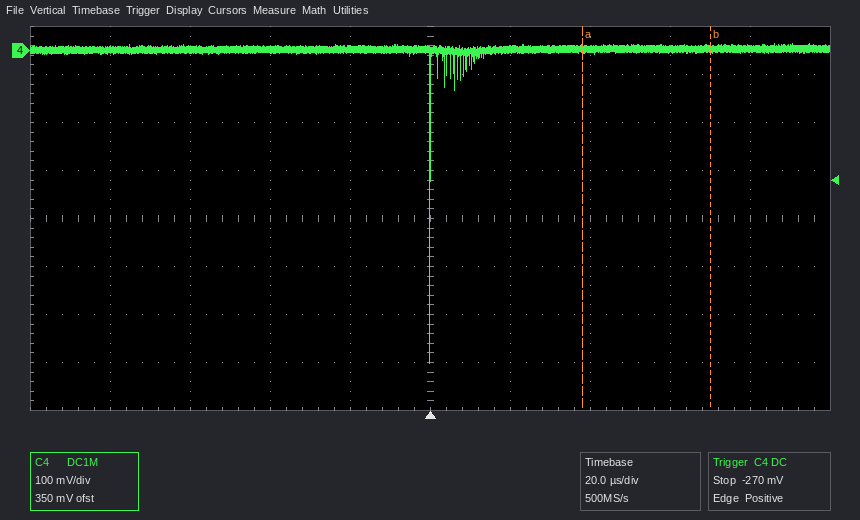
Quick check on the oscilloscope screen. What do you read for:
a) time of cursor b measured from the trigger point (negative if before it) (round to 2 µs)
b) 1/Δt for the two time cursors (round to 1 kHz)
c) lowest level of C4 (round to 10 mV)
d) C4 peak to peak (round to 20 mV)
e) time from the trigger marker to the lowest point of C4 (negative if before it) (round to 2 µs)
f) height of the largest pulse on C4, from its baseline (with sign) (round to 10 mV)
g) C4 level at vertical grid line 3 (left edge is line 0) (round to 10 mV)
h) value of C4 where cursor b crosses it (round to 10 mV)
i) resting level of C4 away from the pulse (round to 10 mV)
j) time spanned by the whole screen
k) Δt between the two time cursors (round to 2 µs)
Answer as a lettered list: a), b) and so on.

a) +70 µs
b) 31 kHz
c) -650 mV
d) 660 mV
e) 0 µs
f) -650 mV
g) 0 mV
h) 0 mV
i) 0 mV
j) 200 µs
k) 32 µs
